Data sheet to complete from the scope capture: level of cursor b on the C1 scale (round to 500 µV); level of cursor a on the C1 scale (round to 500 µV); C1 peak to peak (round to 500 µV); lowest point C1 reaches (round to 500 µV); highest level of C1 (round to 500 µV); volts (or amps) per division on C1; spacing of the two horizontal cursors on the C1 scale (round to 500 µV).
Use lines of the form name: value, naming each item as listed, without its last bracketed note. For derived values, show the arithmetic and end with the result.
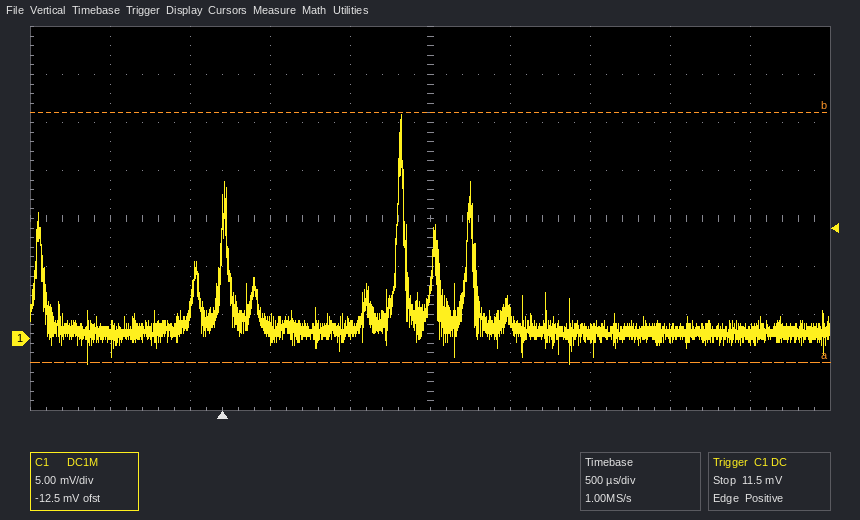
level of cursor b on the C1 scale: 23.5 mV
level of cursor a on the C1 scale: -2.5 mV
C1 peak to peak: 23.5 mV − (-2.5 mV) = 26.0 mV
lowest point C1 reaches: -2.5 mV
highest level of C1: 23.5 mV
volts (or amps) per division on C1: 5 mV
spacing of the two horizontal cursors on the C1 scale: 26.0 mV
